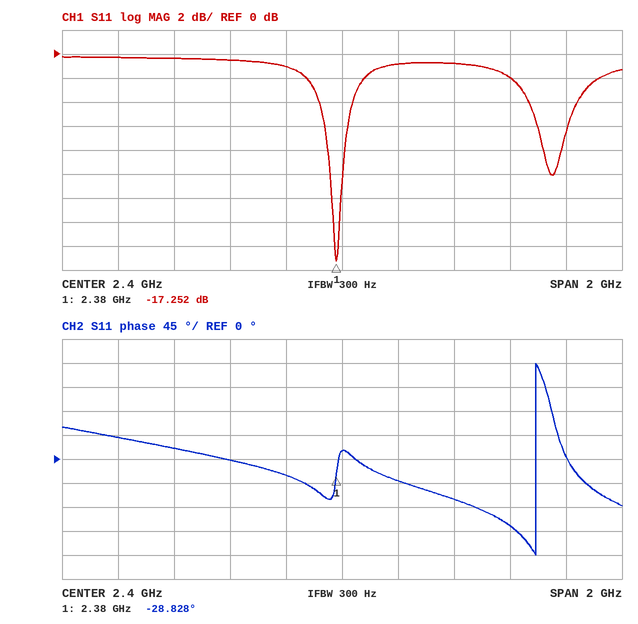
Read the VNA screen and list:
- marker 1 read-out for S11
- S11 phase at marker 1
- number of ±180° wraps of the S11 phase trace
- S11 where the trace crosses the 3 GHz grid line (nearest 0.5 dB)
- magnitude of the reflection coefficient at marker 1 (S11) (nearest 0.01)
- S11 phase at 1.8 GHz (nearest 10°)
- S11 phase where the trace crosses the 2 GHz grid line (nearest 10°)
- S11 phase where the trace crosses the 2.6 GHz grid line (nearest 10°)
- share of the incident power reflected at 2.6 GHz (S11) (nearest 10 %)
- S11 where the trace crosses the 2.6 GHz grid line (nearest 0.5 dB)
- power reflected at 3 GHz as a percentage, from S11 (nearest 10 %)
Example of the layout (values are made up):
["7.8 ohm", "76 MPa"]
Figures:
["-17.252 dB", "-28.828°", "1", "-2.0 dB", "0.14", "20°", "0°", "-40°", "80 %", "-1.0 dB", "60 %"]
